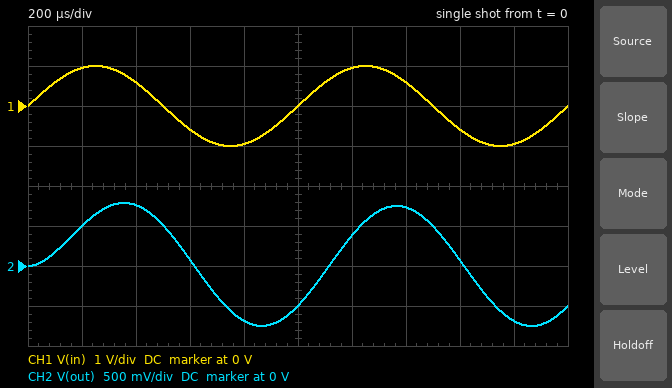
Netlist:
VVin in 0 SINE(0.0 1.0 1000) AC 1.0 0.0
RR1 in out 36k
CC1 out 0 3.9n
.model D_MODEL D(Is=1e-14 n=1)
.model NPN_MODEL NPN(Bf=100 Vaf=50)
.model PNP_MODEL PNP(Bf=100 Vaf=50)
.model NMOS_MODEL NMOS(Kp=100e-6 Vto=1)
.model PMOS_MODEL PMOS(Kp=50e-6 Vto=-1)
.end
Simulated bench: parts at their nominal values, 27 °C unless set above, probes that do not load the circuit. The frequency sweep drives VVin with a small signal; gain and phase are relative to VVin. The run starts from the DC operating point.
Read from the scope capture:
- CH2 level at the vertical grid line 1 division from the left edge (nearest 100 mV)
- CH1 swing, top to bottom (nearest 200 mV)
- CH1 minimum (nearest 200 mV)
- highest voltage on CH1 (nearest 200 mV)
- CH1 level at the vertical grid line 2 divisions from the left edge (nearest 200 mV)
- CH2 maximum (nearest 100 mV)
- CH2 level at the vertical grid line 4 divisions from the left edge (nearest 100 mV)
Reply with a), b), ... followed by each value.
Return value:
a) 500 mV
b) 2.0 V
c) -1.0 V
d) 1.0 V
e) 600 mV
f) 800 mV
g) -700 mV
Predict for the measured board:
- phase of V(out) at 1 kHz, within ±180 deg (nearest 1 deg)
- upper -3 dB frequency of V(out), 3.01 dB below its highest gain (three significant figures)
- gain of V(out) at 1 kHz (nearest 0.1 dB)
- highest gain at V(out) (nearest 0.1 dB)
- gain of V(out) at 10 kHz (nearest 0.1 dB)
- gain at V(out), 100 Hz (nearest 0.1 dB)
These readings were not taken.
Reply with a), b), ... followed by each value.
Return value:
a) -41 deg
b) 1.13 kHz
c) -2.5 dB
d) 0 dB
e) -19.0 dB
f) 0 dB
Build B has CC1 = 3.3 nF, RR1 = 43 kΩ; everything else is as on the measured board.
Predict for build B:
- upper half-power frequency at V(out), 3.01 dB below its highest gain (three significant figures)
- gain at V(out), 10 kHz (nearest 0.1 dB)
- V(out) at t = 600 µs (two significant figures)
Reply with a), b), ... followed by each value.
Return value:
a) 1.12 kHz
b) -19.1 dB
c) 82 mV
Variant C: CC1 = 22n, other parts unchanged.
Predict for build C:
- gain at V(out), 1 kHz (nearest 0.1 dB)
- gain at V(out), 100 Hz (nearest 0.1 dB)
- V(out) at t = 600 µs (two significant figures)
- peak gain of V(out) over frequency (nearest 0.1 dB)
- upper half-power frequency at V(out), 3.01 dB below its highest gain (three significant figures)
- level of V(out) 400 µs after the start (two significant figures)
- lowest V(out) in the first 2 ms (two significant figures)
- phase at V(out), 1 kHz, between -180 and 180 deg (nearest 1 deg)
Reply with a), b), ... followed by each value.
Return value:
a) -14.1 dB
b) -1.0 dB
c) 220 mV
d) 0 dB
e) 201 Hz
f) 300 mV
g) -180 mV
h) -79 deg
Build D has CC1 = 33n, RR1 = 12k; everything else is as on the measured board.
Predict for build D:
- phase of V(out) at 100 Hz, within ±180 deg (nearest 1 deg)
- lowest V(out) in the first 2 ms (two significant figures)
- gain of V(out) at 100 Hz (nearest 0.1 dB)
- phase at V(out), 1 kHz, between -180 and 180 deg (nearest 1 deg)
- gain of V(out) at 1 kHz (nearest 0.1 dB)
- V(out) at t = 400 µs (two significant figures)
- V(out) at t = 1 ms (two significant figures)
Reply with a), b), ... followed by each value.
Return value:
a) -14 deg
b) -370 mV
c) -0.3 dB
d) -68 deg
e) -8.6 dB
f) 490 mV
g) -320 mV
